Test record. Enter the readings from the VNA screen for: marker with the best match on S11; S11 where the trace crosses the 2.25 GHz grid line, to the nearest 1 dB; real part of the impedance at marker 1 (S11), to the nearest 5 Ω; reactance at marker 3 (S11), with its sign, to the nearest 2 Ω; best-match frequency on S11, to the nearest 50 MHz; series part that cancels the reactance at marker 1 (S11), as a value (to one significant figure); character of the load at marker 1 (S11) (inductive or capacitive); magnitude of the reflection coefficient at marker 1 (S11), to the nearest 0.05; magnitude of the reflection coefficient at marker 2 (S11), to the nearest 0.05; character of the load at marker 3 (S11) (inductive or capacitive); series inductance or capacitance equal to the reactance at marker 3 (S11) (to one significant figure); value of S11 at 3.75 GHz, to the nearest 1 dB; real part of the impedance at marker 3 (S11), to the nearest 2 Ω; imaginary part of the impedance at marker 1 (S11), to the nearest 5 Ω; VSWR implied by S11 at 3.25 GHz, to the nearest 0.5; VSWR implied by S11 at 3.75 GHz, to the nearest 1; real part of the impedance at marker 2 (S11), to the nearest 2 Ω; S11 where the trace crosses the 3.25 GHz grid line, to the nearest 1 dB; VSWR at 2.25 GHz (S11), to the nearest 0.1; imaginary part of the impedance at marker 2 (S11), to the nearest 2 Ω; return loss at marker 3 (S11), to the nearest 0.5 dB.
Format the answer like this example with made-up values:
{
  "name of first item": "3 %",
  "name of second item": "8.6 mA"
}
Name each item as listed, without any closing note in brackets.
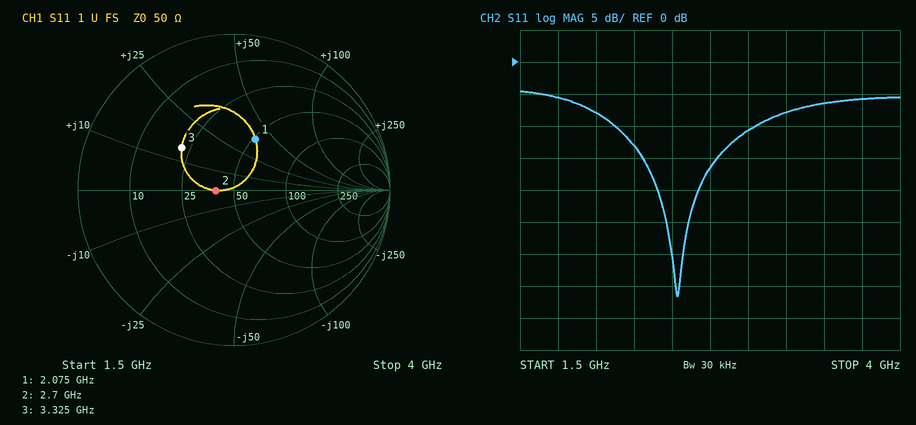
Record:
{
  "marker with the best match on S11": "marker 2",
  "S11 where the trace crosses the 2.25 GHz grid line, to the nearest 1 dB": "-13 dB",
  "real part of the impedance at marker 1 (S11), to the nearest 5 Ω": "50 Ω",
  "reactance at marker 3 (S11), with its sign, to the nearest 2 Ω": "+14 Ω",
  "best-match frequency on S11, to the nearest 50 MHz": "2.55 GHz",
  "series part that cancels the reactance at marker 1 (S11), as a value": "2 pF",
  "character of the load at marker 1 (S11)": "inductive",
  "magnitude of the reflection coefficient at marker 1 (S11), to the nearest 0.05": "0.35",
  "magnitude of the reflection coefficient at marker 2 (S11), to the nearest 0.05": "0.10",
  "character of the load at marker 3 (S11)": "inductive",
  "series inductance or capacitance equal to the reactance at marker 3 (S11)": "700 pH",
  "value of S11 at 3.75 GHz, to the nearest 1 dB": "-6 dB",
  "real part of the impedance at marker 3 (S11), to the nearest 2 Ω": "22 Ω",
  "imaginary part of the impedance at marker 1 (S11), to the nearest 5 Ω": "+40 Ω",
  "VSWR implied by S11 at 3.25 GHz, to the nearest 0.5": "2.5",
  "VSWR implied by S11 at 3.75 GHz, to the nearest 1": "3",
  "real part of the impedance at marker 2 (S11), to the nearest 2 Ω": "40 Ω",
  "S11 where the trace crosses the 3.25 GHz grid line, to the nearest 1 dB": "-8 dB",
  "VSWR at 2.25 GHz (S11), to the nearest 0.1": "1.6",
  "imaginary part of the impedance at marker 2 (S11), to the nearest 2 Ω": "0 Ω",
  "return loss at marker 3 (S11), to the nearest 0.5 dB": "7.5 dB"
}
